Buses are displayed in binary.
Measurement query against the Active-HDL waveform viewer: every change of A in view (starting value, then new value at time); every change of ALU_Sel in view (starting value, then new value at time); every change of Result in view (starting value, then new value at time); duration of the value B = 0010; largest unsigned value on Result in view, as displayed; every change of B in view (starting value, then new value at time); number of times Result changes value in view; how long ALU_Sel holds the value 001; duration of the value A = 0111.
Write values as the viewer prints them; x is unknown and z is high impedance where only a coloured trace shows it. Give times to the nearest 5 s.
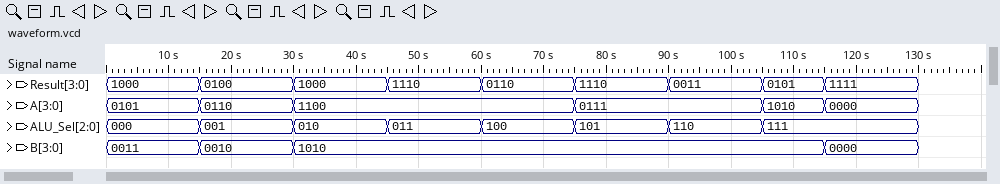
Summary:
0101, 0110 at 15 s, 1100 at 30 s, 0111 at 75 s, 1010 at 105 s, 0000 at 115 s
000, 001 at 15 s, 010 at 30 s, 011 at 45 s, 100 at 60 s, 101 at 75 s, 110 at 90 s, 111 at 105 s
1000, 0100 at 15 s, 1000 at 30 s, 1110 at 45 s, 0110 at 60 s, 1110 at 75 s, 0011 at 90 s, 0101 at 105 s, 1111 at 115 s
15 s
1111
0011, 0010 at 15 s, 1010 at 30 s, 0000 at 115 s
8
15 s
30 s
